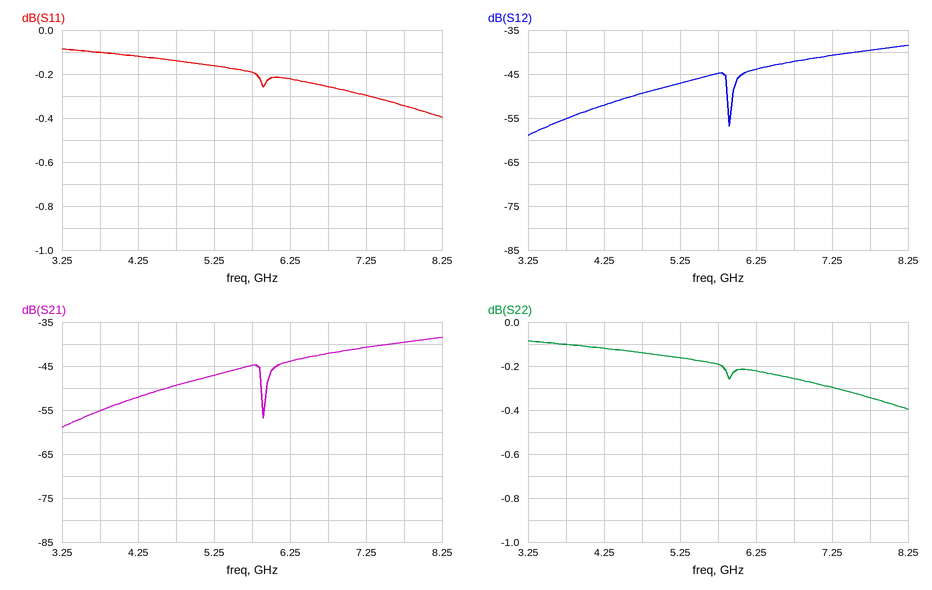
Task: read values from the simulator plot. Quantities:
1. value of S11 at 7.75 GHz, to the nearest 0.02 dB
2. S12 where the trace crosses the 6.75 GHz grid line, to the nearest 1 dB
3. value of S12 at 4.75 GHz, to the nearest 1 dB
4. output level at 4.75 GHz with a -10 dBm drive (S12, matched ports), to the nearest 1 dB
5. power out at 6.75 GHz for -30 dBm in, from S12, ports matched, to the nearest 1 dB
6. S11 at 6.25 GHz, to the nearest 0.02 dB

-0.34 dB
-42 dB
-49 dB
-59 dBm
-72 dBm
-0.22 dB
